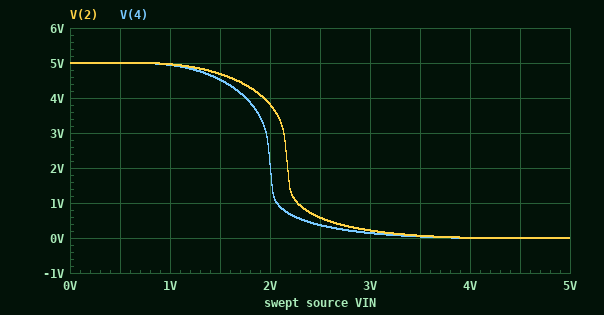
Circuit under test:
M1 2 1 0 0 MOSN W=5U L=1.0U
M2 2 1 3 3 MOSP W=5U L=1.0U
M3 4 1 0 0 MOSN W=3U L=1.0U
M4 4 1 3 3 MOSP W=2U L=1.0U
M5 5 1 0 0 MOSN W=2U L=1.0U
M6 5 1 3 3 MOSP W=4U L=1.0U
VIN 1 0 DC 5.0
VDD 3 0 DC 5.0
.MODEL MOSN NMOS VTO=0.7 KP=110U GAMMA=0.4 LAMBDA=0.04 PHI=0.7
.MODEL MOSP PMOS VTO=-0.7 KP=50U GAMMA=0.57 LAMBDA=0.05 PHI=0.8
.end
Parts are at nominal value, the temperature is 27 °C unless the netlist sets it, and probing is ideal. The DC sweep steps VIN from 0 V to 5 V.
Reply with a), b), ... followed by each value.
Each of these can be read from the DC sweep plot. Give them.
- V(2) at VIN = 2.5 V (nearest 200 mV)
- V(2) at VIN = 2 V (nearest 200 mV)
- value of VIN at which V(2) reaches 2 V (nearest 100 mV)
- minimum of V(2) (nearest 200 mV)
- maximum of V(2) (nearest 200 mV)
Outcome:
a) 600 mV
b) 3.8 V
c) 2.2 V
d) 0 V
e) 5.0 V
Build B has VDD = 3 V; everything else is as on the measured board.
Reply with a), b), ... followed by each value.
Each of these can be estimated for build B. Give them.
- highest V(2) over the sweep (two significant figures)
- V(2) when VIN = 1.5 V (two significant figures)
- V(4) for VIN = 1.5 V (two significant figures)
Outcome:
a) 3.0 V
b) 240 mV
c) 150 mV
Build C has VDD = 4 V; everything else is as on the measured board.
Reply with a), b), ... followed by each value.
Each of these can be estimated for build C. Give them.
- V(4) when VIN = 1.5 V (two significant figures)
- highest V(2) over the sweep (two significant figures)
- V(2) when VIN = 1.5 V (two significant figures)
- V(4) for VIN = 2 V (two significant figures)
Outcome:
a) 3.2 V
b) 4.0 V
c) 3.5 V
d) 260 mV
